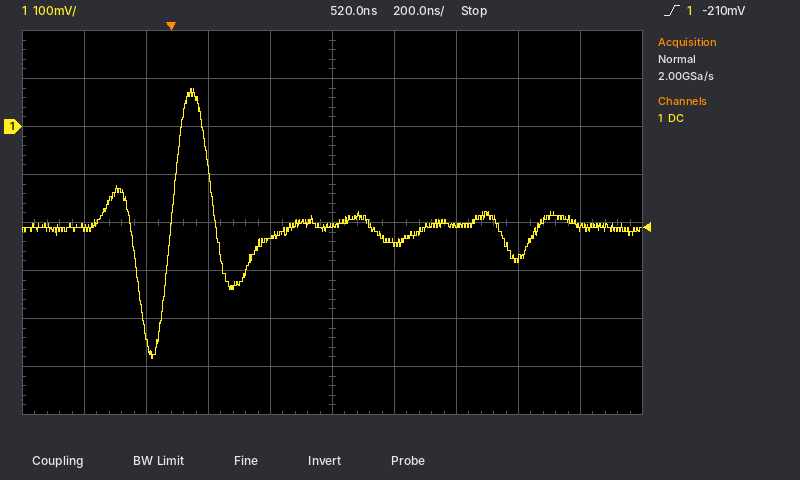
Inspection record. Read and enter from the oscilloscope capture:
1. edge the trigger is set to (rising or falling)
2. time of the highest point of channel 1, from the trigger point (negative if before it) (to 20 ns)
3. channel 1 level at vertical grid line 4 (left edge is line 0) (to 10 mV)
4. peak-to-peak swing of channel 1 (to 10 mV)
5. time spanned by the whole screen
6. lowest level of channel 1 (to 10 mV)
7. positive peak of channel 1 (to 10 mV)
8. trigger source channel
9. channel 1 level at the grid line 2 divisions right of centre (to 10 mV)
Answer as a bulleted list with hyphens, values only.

- rising
- +60 ns
- -230 mV
- 560 mV
- 2 µs
- -480 mV
- 80 mV
- channel 1
- -210 mV
